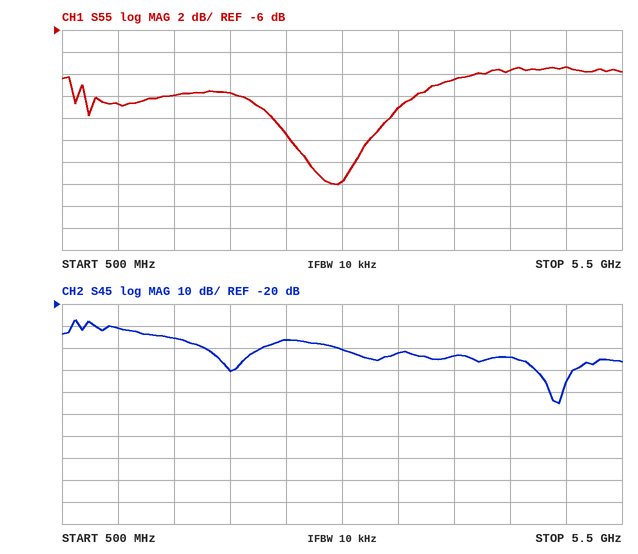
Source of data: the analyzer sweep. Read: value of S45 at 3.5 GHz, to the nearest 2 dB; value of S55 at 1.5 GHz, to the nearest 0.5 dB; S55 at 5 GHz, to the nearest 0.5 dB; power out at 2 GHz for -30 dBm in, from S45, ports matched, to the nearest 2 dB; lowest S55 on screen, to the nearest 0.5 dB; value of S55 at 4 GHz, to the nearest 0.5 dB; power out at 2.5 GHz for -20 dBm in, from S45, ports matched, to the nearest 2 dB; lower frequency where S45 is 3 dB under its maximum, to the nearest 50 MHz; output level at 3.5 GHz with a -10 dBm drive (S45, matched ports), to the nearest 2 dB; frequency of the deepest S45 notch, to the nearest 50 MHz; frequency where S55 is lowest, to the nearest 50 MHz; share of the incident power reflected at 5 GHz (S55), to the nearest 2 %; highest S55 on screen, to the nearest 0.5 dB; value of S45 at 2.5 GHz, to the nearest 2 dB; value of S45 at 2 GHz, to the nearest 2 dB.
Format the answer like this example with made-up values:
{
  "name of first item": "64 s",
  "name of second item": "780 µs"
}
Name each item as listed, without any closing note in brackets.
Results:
{
  "value of S45 at 3.5 GHz, to the nearest 2 dB": "-42 dB",
  "value of S55 at 1.5 GHz, to the nearest 0.5 dB": "-12.0 dB",
  "S55 at 5 GHz, to the nearest 0.5 dB": "-9.5 dB",
  "power out at 2 GHz for -30 dBm in, from S45, ports matched, to the nearest 2 dB": "-80 dBm",
  "lowest S55 on screen, to the nearest 0.5 dB": "-20.0 dB",
  "value of S55 at 4 GHz, to the nearest 0.5 dB": "-10.5 dB",
  "power out at 2.5 GHz for -20 dBm in, from S45, ports matched, to the nearest 2 dB": "-56 dBm",
  "lower frequency where S45 is 3 dB under its maximum, to the nearest 50 MHz": "600 MHz",
  "output level at 3.5 GHz with a -10 dBm drive (S45, matched ports), to the nearest 2 dB": "-52 dBm",
  "frequency of the deepest S45 notch, to the nearest 50 MHz": "4.95 GHz",
  "frequency where S55 is lowest, to the nearest 50 MHz": "2.95 GHz",
  "share of the incident power reflected at 5 GHz (S55), to the nearest 2 %": "12 %",
  "highest S55 on screen, to the nearest 0.5 dB": "-9.5 dB",
  "value of S45 at 2.5 GHz, to the nearest 2 dB": "-36 dB",
  "value of S45 at 2 GHz, to the nearest 2 dB": "-50 dB"
}
